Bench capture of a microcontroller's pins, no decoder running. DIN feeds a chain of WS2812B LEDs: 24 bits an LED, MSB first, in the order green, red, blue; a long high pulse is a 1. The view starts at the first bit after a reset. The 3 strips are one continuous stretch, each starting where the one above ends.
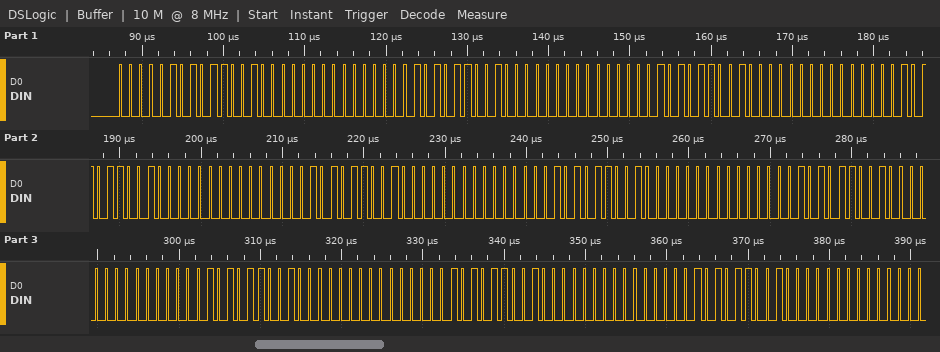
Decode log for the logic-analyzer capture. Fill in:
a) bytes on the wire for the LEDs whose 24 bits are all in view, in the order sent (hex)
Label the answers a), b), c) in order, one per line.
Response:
a) 05 64 00 05 64 00 05 64 00 05 64 00 05 64 00 05 64 00 05 64 00 05 64 00 05 64 00 05 64 00
